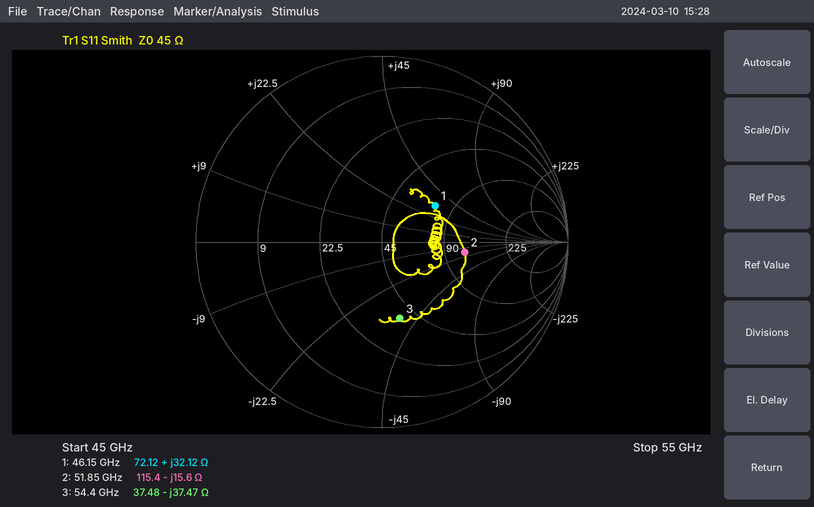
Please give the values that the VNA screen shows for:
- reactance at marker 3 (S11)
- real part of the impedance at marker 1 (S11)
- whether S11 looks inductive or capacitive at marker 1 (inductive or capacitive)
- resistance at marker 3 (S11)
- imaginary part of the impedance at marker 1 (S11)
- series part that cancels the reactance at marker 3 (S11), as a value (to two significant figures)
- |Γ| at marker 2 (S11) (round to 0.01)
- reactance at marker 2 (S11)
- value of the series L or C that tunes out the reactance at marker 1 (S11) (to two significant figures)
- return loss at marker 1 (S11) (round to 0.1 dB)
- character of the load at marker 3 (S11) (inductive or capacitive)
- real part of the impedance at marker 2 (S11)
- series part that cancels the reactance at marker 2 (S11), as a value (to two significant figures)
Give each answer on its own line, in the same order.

-37.47 Ω
72.12 Ω
inductive
37.48 Ω
+32.12 Ω
110 pH
0.45
-15.6 Ω
110 fF
9.2 dB
capacitive
115.4 Ω
48 pH
